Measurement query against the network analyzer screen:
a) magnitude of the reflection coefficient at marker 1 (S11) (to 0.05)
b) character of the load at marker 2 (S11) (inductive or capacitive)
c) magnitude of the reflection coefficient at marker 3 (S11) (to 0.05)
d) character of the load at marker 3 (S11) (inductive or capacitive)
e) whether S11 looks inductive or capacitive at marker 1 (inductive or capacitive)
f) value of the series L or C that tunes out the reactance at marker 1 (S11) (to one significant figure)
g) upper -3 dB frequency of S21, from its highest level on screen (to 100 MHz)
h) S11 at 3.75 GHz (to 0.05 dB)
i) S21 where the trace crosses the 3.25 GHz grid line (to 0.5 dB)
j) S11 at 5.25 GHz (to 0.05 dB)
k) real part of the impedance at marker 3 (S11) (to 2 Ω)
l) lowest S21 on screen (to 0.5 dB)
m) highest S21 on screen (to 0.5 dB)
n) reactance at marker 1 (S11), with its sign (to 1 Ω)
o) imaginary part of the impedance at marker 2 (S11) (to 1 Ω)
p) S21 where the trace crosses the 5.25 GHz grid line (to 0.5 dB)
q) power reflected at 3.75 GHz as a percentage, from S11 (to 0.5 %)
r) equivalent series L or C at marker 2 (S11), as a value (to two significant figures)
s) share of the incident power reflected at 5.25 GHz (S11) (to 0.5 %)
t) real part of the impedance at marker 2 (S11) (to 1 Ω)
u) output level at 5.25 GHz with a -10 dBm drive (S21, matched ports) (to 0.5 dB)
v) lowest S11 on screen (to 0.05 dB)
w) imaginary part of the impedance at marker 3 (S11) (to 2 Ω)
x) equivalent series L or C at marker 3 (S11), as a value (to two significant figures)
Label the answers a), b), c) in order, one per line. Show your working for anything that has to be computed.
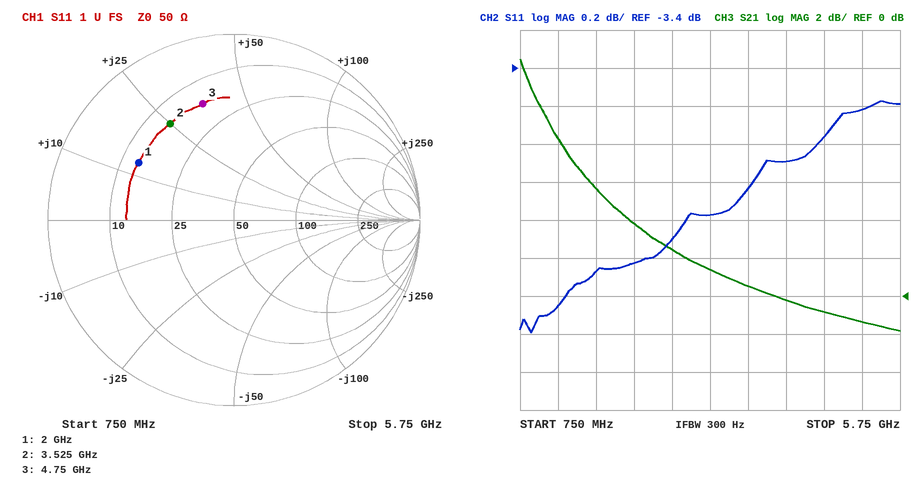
a) 0.60
b) inductive
c) 0.65
d) inductive
e) inductive
f) C = 1/(2π × 2 GHz × 13 Ω) ≈ 6 pF
g) 1.1 GHz
h) -4.05 dB
i) 1.5 dB
j) -3.60 dB
k) 16 Ω
l) -2.0 dB
m) 12.5 dB
n) +13 Ω
o) +25 Ω
p) -1.5 dB
q) 10^(-4.05/10) ≈ 39.4 %, so 39.5 % to the nearest 0.5 %
r) L = 25 Ω/(2π × 3.525 GHz) ≈ 1.1 nH
s) 10^(-3.6/10) ≈ 43.7 %, so 43.5 % to the nearest 0.5 %
t) 15 Ω
u) -10 dBm + (-1.5 dB) = -11.5 dBm
v) -4.80 dB
w) +36 Ω
x) L = 36 Ω/(2π × 4.75 GHz) ≈ 1.2 nH
